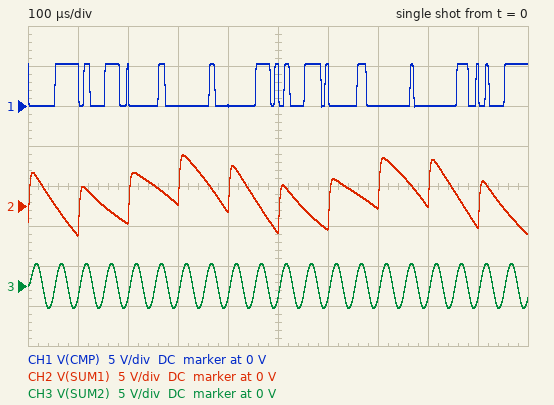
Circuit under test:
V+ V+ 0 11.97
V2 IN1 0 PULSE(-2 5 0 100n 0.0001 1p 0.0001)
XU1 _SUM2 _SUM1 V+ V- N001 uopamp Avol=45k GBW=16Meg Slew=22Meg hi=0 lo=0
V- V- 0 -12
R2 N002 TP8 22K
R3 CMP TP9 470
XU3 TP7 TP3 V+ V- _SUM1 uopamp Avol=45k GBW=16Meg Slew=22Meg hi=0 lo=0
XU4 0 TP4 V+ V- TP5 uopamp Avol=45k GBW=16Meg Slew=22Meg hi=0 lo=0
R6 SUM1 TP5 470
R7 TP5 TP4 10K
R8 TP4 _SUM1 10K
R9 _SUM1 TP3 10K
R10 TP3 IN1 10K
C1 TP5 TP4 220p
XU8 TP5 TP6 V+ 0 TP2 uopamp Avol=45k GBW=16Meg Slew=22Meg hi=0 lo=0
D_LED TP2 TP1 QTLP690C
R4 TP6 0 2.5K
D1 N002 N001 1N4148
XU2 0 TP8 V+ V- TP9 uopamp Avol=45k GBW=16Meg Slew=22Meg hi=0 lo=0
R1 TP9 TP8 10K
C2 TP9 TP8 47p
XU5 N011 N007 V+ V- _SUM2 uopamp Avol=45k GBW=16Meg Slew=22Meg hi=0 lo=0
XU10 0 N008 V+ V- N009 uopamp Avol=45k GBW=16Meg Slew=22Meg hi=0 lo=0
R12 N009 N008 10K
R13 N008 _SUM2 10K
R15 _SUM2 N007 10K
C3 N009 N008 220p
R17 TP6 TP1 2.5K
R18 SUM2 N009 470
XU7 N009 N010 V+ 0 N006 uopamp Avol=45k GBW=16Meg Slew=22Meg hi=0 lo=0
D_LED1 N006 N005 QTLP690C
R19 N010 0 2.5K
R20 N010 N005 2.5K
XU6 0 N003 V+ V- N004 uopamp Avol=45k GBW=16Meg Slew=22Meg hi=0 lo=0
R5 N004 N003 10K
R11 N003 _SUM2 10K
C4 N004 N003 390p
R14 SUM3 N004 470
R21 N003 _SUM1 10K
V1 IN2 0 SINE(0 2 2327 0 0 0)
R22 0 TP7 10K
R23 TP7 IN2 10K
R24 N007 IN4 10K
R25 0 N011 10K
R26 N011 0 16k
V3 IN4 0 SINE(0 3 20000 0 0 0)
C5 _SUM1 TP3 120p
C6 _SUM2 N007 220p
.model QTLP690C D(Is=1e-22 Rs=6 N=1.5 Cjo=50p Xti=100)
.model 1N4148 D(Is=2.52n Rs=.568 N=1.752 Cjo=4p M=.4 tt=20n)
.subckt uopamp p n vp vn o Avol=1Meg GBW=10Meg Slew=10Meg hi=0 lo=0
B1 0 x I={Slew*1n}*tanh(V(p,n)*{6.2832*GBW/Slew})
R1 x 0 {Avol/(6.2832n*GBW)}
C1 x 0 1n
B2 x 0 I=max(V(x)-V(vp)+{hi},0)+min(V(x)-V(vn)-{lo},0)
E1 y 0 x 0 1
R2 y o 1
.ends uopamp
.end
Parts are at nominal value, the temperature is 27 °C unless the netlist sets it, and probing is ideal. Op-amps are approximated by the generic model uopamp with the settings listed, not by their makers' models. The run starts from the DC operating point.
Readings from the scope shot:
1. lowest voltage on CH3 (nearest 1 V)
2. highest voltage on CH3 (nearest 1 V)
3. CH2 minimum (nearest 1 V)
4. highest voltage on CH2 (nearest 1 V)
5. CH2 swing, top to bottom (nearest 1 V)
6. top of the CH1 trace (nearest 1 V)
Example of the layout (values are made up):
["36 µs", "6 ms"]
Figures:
["-3 V", "3 V", "-4 V", "6 V", "10 V", "5 V"]
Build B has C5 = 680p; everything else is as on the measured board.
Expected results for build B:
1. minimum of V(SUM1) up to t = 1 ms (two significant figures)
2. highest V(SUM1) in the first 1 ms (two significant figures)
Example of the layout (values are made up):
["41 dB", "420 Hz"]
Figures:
["-3.3 V", "5.7 V"]
